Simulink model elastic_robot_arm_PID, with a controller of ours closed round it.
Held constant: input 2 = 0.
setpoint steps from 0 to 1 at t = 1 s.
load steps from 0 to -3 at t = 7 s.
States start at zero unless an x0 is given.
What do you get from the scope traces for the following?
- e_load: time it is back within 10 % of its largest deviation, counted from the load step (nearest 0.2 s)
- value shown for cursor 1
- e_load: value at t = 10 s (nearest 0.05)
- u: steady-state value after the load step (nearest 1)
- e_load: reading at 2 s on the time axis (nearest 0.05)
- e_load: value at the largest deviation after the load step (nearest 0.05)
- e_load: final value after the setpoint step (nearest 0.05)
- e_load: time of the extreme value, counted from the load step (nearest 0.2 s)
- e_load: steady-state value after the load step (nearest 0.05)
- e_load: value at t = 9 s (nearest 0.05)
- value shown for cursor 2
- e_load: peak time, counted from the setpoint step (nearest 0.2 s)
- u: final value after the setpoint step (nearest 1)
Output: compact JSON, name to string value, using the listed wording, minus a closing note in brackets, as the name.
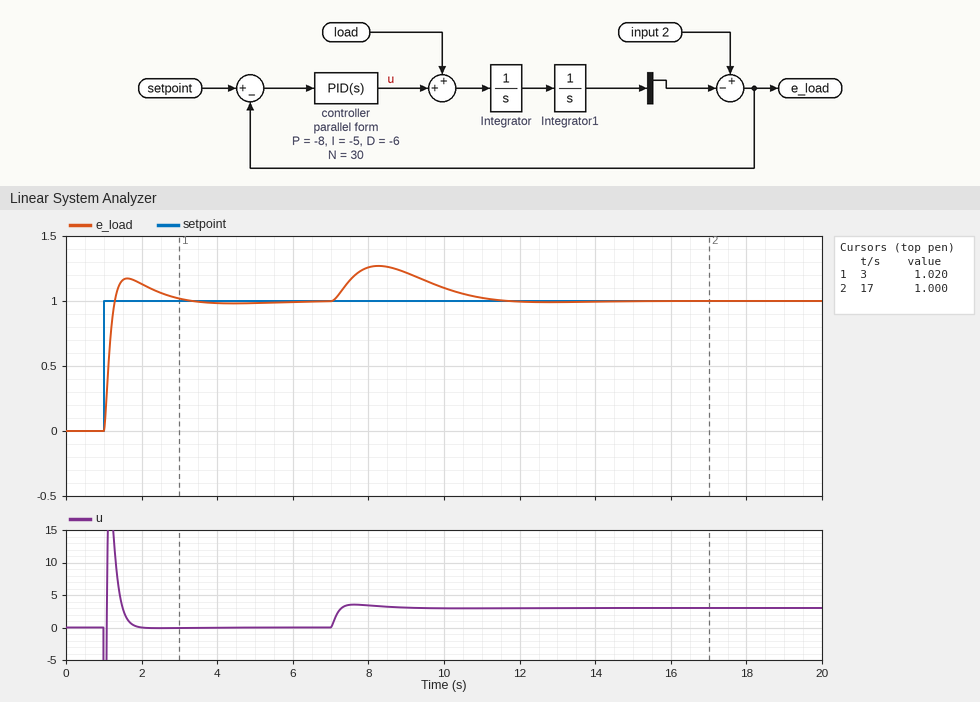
{"e_load: time it is back within 10 % of its largest deviation, counted from the load step": "4.0 s", "value shown for cursor 1": "1.020", "e_load: value at t = 10 s": "1.10", "u: steady-state value after the load step": "3", "e_load: reading at 2 s on the time axis": "1.15", "e_load: value at the largest deviation after the load step": "1.25", "e_load: final value after the setpoint step": "1.00", "e_load: time of the extreme value, counted from the load step": "1.2 s", "e_load: steady-state value after the load step": "1.00", "e_load: value at t = 9 s": "1.20", "value shown for cursor 2": "1.000", "e_load: peak time, counted from the setpoint step": "0.6 s", "u: final value after the setpoint step": "0"}
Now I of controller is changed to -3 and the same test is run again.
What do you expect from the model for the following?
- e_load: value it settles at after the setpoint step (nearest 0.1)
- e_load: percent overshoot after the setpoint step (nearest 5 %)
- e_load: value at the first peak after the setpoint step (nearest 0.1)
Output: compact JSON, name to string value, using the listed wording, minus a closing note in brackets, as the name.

{"e_load: value it settles at after the setpoint step": "1.0", "e_load: percent overshoot after the setpoint step": "15 %", "e_load: value at the first peak after the setpoint step": "1.2"}
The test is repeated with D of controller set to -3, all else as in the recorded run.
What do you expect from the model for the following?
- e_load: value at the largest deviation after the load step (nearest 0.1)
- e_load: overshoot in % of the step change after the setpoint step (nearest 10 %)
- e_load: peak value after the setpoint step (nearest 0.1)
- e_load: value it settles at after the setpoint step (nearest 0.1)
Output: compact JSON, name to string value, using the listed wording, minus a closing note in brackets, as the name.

{"e_load: value at the largest deviation after the load step": "1.4", "e_load: overshoot in % of the step change after the setpoint step": "40 %", "e_load: peak value after the setpoint step": "1.4", "e_load: value it settles at after the setpoint step": "1.0"}
